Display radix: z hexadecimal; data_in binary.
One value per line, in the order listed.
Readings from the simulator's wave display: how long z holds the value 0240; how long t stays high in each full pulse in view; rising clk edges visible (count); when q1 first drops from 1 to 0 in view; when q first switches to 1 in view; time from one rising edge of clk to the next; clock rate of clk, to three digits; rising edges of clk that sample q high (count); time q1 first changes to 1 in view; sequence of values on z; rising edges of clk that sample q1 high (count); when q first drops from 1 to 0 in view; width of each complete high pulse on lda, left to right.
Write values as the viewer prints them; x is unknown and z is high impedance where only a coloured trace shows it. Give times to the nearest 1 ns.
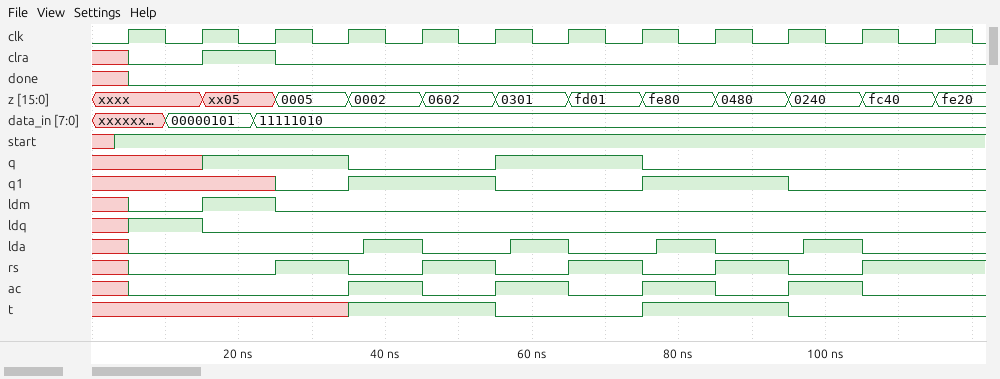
10 ns
20 ns
12
55 ns
15 ns
10 ns
100 MHz
4
35 ns
xxxx, xx05, 0005, 0002, 0602, 0301, fd01, fe80, 0480, 0240, fc40, fe20
4
35 ns
8 ns, 8 ns, 8 ns, 8 ns
